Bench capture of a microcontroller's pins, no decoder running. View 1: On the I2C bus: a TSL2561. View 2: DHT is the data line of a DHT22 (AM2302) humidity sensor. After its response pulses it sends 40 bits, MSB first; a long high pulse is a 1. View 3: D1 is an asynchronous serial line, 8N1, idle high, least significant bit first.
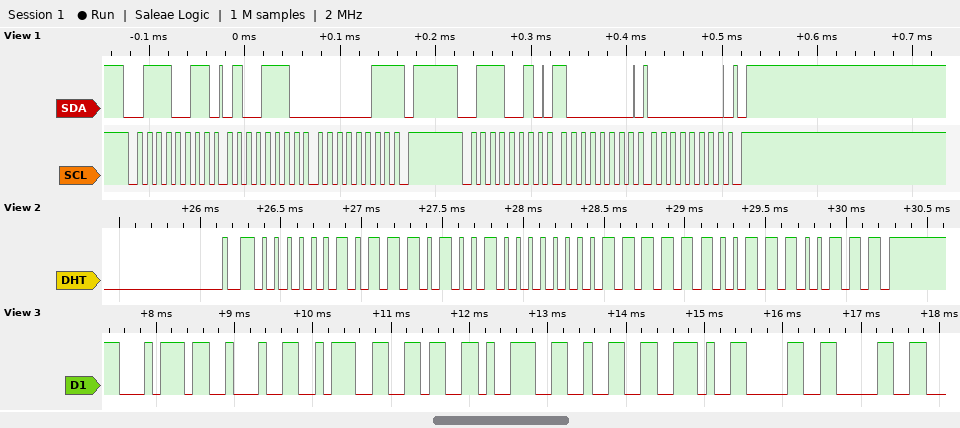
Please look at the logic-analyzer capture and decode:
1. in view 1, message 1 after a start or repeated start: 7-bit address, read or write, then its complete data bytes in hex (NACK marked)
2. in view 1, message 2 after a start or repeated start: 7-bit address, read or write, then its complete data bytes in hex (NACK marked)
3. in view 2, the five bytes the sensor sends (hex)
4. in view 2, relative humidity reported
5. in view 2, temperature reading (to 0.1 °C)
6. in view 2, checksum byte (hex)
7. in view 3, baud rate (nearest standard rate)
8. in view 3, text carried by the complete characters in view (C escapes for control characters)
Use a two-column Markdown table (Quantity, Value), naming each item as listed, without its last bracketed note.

| Quantity | Value |
|---|---|
| in view 1, message 1 after a start or repeated start: 7-bit address, read or write, then its complete data bytes in hex | 0x39 read: 4E 03 NACK |
| in view 1, message 2 after a start or repeated start: 7-bit address, read or write, then its complete data bytes in hex | 0x39 write: 80 00 |
| in view 2, the five bytes the sensor sends | 02 E9 00 FC E7 |
| in view 2, relative humidity reported | 74.5 % |
| in view 2, temperature reading | 25.2 °C |
| in view 2, checksum byte | 0xE7 |
| in view 3, baud rate | 9600 baud |
| in view 3, text carried by the complete characters in view | "t\":692.00" |
